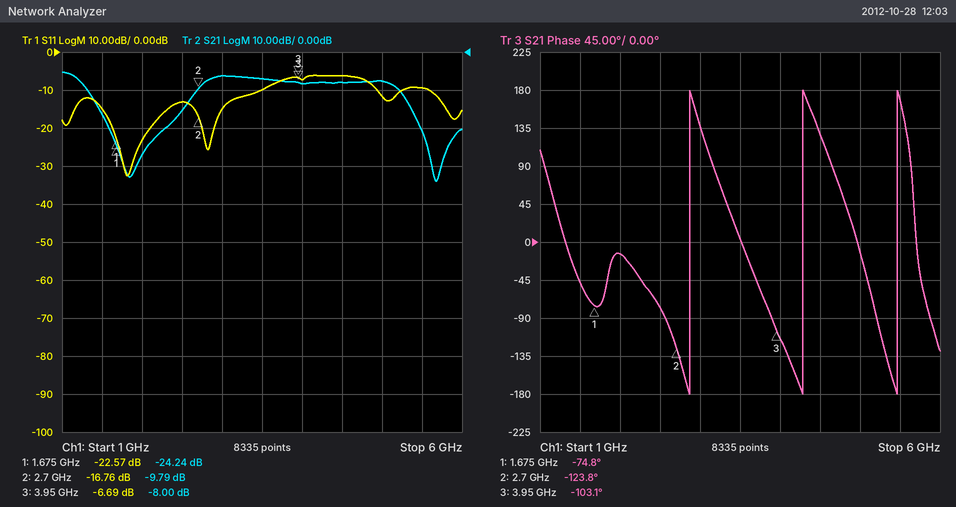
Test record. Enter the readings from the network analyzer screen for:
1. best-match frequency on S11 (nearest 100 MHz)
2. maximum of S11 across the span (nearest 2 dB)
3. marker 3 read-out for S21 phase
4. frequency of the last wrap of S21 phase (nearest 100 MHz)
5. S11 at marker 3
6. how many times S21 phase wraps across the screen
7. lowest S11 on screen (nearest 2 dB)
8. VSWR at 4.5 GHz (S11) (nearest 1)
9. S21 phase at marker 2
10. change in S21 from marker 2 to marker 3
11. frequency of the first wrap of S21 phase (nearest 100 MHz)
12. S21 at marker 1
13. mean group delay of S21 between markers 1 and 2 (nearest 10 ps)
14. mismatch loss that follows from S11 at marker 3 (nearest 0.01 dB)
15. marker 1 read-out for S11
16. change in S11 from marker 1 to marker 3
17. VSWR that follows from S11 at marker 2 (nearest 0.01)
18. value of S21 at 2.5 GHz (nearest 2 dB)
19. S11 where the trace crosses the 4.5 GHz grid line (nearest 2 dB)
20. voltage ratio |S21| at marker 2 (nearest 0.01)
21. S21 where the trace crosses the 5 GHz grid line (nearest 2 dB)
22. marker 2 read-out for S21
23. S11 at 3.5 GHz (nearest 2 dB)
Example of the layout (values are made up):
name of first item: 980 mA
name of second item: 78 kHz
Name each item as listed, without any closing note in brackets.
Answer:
best-match frequency on S11: 1.8 GHz
maximum of S11 across the span: -6 dB
marker 3 read-out for S21 phase: -103.1°
frequency of the last wrap of S21 phase: 5.5 GHz
S11 at marker 3: -6.69 dB
how many times S21 phase wraps across the screen: 3
lowest S11 on screen: -32 dB
VSWR at 4.5 GHz (S11): 3
S21 phase at marker 2: -123.8°
change in S21 from marker 2 to marker 3: 1.79 dB
frequency of the first wrap of S21 phase: 2.9 GHz
S21 at marker 1: -24.24 dB
mean group delay of S21 between markers 1 and 2: 130 ps
mismatch loss that follows from S11 at marker 3: 1.05 dB
marker 1 read-out for S11: -22.57 dB
change in S11 from marker 1 to marker 3: 15.88 dB
VSWR that follows from S11 at marker 2: 1.34
value of S21 at 2.5 GHz: -16 dB
S11 where the trace crosses the 4.5 GHz grid line: -6 dB
voltage ratio |S21| at marker 2: 0.32
S21 where the trace crosses the 5 GHz grid line: -8 dB
marker 2 read-out for S21: -9.79 dB
S11 at 3.5 GHz: -10 dB
